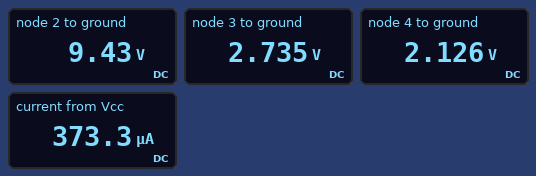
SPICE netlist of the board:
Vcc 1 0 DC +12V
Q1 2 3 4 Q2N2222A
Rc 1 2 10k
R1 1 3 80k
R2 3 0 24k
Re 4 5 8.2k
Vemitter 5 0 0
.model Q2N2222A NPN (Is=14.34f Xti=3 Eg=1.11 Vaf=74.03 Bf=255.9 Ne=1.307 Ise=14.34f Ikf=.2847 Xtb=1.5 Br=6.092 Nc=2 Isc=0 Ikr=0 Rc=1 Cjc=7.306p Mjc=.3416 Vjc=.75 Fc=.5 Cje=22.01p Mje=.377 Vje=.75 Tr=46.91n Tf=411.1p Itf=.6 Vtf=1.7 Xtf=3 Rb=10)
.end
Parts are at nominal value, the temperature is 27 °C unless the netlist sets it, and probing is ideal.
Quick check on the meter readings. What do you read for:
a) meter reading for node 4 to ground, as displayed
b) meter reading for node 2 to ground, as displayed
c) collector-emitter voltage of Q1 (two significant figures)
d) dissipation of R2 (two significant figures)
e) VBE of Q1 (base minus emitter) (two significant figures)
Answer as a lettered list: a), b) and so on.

a) 2.126 V
b) 9.43 V
c) 7.3 V
d) 310 µW
e) 610 mV
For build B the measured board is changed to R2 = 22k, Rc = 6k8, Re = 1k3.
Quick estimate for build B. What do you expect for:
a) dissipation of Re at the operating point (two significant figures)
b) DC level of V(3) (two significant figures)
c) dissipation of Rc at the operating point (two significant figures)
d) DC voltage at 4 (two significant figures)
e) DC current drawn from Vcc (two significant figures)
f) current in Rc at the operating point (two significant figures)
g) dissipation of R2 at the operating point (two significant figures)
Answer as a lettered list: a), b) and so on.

a) 2.4 mW
b) 2.4 V
c) 13 mW
d) 1.8 V
e) 1.5 mA
f) 1.4 mA
g) 270 µW
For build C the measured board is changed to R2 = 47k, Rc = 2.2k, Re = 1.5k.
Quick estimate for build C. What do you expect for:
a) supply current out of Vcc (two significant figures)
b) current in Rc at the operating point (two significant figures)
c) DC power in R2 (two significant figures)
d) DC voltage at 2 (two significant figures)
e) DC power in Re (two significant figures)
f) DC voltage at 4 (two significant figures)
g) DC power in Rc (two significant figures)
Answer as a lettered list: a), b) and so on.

a) 2.3 mA
b) 2.2 mA
c) 350 µW
d) 7.1 V
e) 7.6 mW
f) 3.4 V
g) 11 mW
